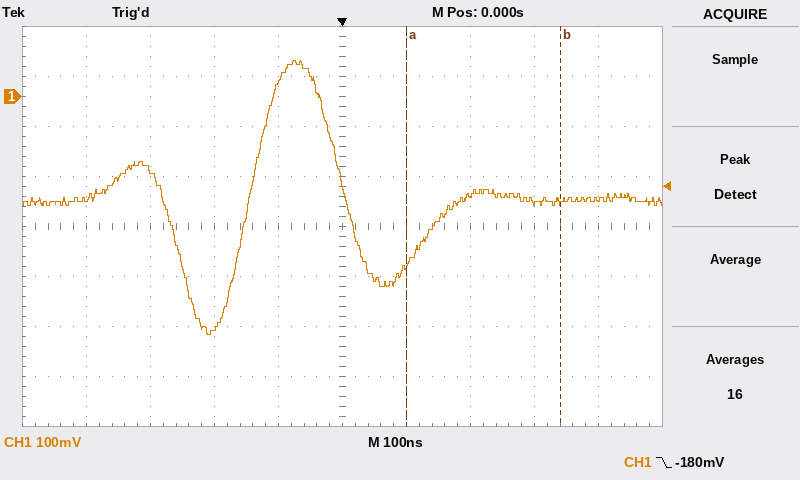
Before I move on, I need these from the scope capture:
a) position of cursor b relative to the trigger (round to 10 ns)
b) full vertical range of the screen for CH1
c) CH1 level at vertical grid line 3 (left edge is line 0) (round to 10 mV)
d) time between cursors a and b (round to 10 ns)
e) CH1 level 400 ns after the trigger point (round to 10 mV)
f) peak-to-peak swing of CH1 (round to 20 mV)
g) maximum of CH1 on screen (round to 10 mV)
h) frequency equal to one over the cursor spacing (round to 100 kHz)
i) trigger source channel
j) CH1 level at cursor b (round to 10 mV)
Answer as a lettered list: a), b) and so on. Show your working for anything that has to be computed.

a) +340 ns
b) 800 mV
c) -460 mV
d) 240 ns
e) -210 mV
f) 540 mV
g) 70 mV
h) 1 / 240 ns ≈ 4.2 MHz
i) CH1
j) -210 mV
